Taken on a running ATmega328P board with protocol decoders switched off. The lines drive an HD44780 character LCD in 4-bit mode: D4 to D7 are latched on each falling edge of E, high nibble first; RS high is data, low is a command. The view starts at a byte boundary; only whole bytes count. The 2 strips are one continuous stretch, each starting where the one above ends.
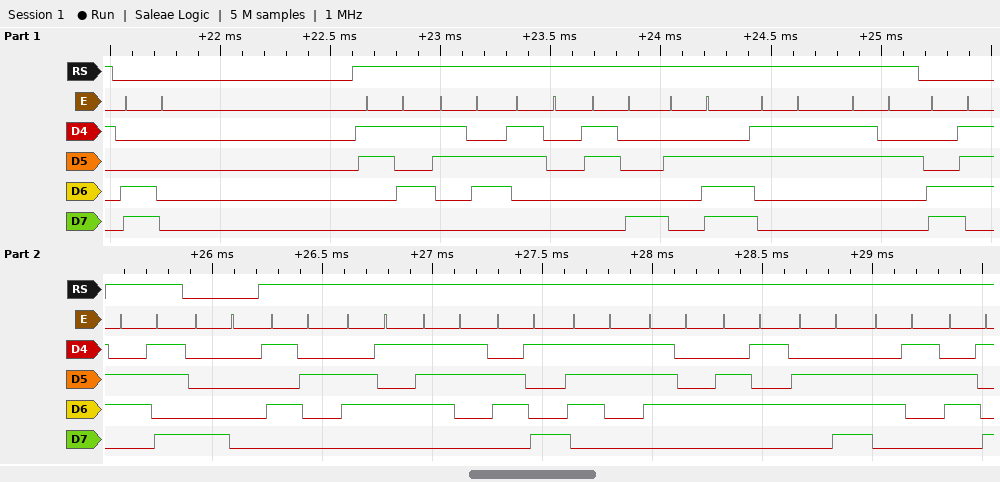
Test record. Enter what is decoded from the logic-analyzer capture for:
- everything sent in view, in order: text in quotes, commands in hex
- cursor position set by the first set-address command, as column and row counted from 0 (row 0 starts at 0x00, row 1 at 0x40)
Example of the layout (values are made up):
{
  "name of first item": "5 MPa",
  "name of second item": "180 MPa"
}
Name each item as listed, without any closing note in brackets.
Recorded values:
{
  "everything sent in view, in order: text in quotes, commands in hex": "0xC0 \"5608.32\" 0xC7 \"k\" 0x80 \"Resistenci\"",
  "cursor position set by the first set-address command, as column and row counted from 0": "column 0, row 1"
}
